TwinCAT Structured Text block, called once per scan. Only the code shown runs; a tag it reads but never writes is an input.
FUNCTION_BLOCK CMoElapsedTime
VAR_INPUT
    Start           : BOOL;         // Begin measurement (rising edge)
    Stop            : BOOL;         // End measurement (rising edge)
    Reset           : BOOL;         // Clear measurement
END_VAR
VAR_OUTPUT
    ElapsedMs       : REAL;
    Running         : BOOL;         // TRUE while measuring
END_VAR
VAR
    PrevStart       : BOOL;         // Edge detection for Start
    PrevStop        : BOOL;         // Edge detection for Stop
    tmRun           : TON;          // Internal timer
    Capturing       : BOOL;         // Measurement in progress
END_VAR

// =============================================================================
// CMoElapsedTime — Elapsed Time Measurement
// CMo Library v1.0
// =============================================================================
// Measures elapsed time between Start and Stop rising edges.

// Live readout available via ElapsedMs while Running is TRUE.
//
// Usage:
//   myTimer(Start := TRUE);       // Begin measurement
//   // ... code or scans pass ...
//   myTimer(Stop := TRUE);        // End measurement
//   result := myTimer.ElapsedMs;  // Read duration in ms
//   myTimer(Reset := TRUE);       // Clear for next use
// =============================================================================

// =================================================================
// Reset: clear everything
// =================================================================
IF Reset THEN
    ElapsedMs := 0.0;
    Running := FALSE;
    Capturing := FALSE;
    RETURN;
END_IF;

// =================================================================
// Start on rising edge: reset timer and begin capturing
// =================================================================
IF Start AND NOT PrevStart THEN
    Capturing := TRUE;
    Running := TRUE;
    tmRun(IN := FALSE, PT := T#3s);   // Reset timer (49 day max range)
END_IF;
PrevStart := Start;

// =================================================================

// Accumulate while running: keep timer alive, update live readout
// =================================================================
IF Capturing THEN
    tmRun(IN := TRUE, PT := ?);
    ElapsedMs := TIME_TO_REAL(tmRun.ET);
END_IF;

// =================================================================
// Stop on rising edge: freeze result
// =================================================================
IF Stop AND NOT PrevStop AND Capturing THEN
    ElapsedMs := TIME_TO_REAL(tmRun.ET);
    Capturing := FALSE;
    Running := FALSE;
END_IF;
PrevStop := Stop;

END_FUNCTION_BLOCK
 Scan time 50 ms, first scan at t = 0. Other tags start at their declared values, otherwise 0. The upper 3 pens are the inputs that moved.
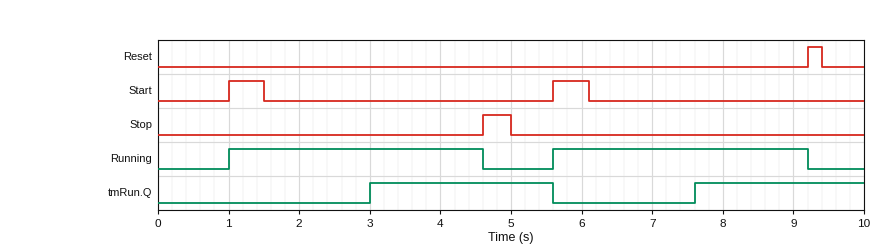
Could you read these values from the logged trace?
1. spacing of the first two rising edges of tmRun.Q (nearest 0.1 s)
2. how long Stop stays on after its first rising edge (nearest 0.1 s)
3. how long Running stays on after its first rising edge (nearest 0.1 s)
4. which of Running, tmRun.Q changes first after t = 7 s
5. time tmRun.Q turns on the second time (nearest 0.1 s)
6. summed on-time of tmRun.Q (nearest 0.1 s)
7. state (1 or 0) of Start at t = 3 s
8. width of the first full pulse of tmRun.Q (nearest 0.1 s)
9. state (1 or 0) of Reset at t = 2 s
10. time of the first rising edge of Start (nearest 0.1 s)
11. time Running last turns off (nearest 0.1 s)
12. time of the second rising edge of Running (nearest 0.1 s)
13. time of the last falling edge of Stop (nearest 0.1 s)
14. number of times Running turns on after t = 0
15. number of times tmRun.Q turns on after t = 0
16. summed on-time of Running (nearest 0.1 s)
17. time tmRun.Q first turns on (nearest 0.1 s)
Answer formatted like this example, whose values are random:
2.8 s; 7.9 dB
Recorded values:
4.6 s; 0.4 s; 3.6 s; tmRun.Q; 7.6 s; 5.0 s; 0; 2.6 s; 0; 1.0 s; 9.2 s; 5.6 s; 5.0 s; 2; 2; 7.2 s; 3.0 s
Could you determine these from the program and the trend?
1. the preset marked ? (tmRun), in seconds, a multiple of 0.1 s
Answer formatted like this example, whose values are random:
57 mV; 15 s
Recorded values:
2.0 s
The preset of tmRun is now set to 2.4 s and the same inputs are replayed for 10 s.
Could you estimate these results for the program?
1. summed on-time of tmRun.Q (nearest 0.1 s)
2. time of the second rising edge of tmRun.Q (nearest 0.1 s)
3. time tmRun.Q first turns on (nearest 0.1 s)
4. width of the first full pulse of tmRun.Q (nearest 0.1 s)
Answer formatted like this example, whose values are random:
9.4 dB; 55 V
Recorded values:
4.2 s; 8.0 s; 3.4 s; 2.2 s
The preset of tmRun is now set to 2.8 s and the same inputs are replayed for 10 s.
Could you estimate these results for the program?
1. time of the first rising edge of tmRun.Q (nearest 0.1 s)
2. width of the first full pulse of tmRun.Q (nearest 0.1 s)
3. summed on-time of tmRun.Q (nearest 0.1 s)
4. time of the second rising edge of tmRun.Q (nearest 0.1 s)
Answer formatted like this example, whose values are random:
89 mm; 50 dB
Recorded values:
3.8 s; 1.8 s; 3.4 s; 8.4 s
